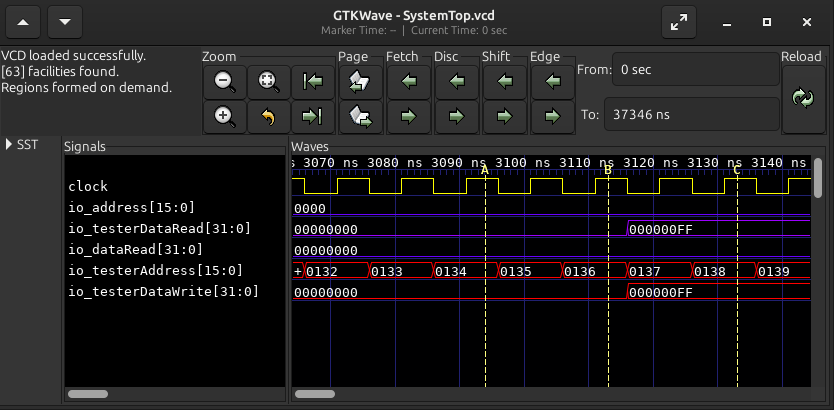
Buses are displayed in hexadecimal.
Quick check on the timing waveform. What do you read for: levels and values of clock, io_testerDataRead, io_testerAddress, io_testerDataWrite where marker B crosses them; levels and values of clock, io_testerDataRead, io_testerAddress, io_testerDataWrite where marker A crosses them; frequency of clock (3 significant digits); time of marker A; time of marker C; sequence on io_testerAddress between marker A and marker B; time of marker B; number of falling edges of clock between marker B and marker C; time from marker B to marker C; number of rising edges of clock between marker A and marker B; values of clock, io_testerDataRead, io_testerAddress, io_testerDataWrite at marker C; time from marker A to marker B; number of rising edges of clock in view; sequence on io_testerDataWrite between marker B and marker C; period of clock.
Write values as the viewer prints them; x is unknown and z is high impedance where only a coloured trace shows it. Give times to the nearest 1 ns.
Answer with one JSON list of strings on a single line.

["clock=1, io_testerDataRead=00000000, io_testerAddress=0136, io_testerDataWrite=00000000", "clock=1, io_testerDataRead=00000000, io_testerAddress=0134, io_testerDataWrite=00000000", "100 MHz", "3094 ns", "3133 ns", "0134, 0135, 0136", "3113 ns", "2", "20 ns", "2", "clock=1, io_testerDataRead=000000FF, io_testerAddress=0138, io_testerDataWrite=000000FF", "19 ns", "8", "00000000, 000000FF", "10 ns"]
